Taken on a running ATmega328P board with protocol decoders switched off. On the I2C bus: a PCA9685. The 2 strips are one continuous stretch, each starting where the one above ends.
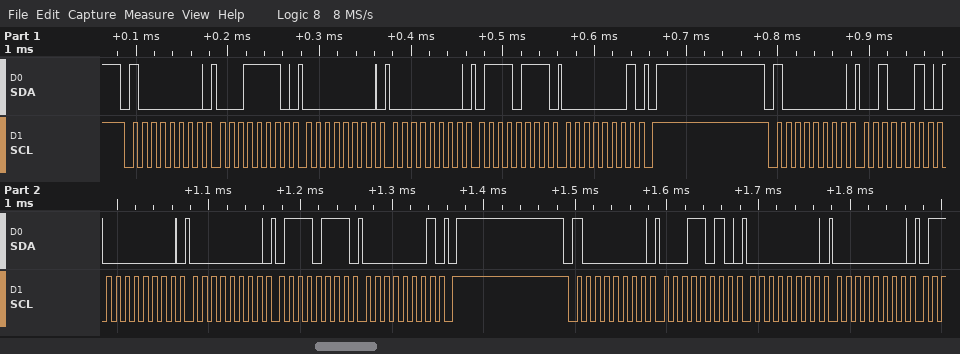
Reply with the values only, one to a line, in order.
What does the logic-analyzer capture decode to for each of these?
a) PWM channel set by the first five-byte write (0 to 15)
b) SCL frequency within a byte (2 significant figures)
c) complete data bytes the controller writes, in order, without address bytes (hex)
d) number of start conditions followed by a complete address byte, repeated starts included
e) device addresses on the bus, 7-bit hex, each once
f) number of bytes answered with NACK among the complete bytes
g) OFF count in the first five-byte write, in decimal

6
100 kHz
1E 00 00 77 01 22 00 00 77 01 1A 00 00
3
0x40
0
375
